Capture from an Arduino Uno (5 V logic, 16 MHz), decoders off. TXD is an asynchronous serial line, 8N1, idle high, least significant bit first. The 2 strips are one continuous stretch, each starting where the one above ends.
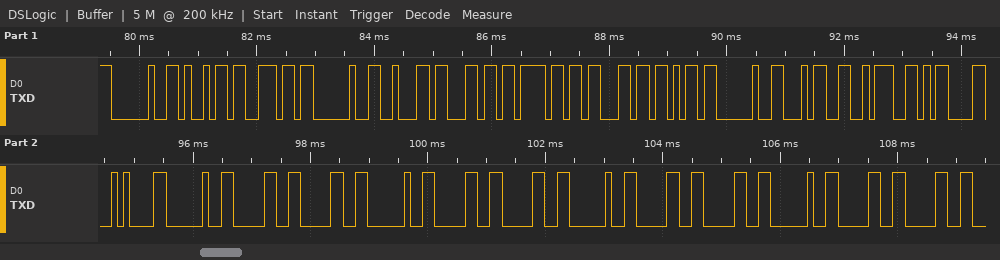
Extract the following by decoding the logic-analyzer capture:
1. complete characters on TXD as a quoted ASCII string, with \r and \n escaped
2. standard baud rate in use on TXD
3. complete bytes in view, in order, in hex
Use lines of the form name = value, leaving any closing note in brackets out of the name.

complete characters on TXD as a quoted ASCII string, with \r and \n escaped = " in block 4:\r\n 00 00 00 00"
standard baud rate in use on TXD = 9600 baud
complete bytes in view, in order, in hex = 0x20 0x69 0x6E 0x20 0x62 0x6C 0x6F 0x63 0x6B 0x20 0x34 0x3A 0x0D 0x0A 0x20 0x30 0x30 0x20 0x30 0x30 0x20 0x30 0x30 0x20 0x30 0x30
